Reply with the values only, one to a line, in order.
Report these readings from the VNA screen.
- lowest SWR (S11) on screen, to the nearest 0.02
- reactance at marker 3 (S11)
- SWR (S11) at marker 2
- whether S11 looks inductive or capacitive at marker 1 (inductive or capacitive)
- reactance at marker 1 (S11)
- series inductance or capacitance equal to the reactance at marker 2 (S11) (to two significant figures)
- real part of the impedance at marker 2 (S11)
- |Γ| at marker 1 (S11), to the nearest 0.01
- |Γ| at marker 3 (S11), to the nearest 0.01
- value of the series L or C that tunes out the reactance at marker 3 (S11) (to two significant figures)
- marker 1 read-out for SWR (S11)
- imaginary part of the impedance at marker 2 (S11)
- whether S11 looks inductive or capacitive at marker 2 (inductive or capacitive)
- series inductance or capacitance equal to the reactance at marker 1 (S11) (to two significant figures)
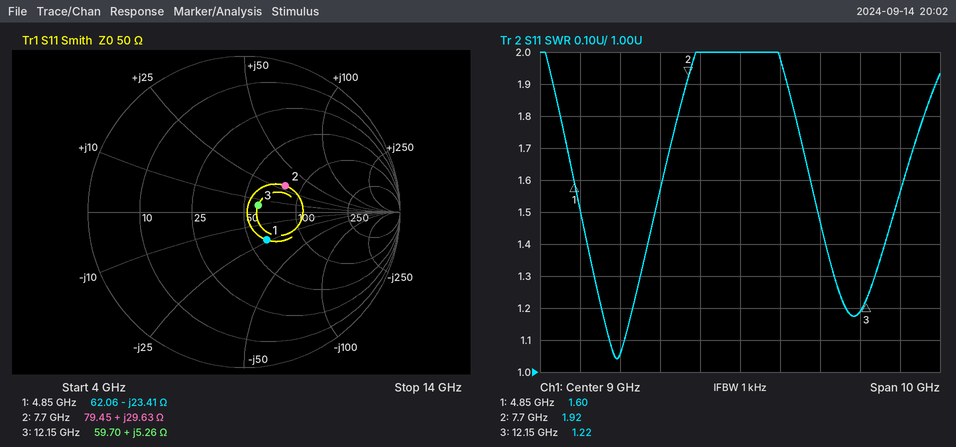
1.04
+5.26 Ω
1.92
capacitive
-23.41 Ω
610 pH
79.45 Ω
0.23
0.10
2.5 pF
1.60
+29.63 Ω
inductive
1.4 pF
